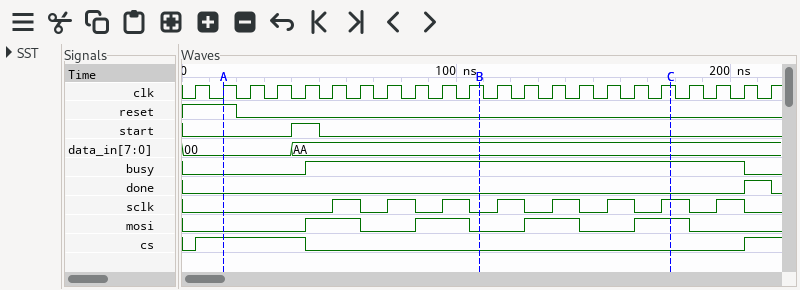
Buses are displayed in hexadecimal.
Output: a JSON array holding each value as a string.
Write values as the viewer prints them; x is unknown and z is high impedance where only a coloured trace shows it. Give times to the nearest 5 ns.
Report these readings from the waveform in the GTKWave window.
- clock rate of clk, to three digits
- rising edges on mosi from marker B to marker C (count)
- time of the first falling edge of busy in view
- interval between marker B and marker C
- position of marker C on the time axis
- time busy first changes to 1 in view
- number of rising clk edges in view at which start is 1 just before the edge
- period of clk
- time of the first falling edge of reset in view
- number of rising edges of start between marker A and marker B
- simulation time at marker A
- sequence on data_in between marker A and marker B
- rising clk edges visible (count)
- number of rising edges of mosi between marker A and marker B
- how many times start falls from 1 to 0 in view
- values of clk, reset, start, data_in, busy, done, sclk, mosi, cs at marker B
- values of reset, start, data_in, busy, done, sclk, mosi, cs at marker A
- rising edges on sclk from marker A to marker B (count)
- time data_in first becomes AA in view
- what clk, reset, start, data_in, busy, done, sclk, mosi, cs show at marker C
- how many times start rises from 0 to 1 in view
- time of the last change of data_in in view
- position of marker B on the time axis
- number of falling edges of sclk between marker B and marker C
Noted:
["100 MHz", "2", "205 ns", "70 ns", "180 ns", "45 ns", "1", "10 ns", "20 ns", "1", "15 ns", "00, AA", "22", "2", "1", "clk=1, reset=0, start=0, data_in=AA, busy=1, done=0, sclk=0, mosi=0, cs=0", "reset=1, start=0, data_in=00, busy=0, done=0, sclk=0, mosi=0, cs=1", "3", "40 ns", "clk=1, reset=0, start=0, data_in=AA, busy=1, done=0, sclk=1, mosi=1, cs=0", "1", "40 ns", "110 ns", "3"]
